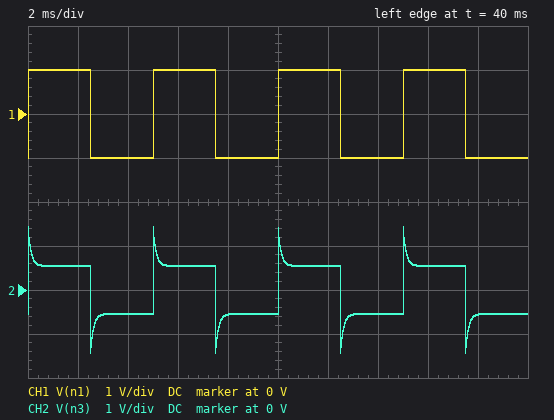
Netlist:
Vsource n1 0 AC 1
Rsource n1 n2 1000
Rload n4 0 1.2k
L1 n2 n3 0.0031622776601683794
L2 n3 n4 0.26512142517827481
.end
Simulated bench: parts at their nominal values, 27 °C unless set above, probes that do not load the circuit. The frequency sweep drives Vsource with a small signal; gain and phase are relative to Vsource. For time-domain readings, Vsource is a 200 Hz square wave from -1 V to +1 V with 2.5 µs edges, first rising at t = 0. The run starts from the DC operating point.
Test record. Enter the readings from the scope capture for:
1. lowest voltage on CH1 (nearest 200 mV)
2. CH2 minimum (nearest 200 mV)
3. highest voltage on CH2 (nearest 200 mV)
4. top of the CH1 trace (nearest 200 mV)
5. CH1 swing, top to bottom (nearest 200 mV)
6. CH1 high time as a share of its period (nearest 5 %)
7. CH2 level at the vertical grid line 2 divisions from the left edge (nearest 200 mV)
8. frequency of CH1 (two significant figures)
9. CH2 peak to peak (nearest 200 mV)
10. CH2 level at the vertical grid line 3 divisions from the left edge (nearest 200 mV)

-1.0 V
-1.4 V
1.4 V
1.0 V
2.0 V
50 %
-600 mV
200 Hz
2.8 V
600 mV
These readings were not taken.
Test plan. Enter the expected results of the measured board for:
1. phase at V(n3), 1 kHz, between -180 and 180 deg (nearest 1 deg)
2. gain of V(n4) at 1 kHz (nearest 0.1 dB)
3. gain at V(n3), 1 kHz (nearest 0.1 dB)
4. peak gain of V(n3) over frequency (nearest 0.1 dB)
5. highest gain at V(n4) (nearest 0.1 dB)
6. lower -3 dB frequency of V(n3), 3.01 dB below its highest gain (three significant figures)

17 deg
-7.3 dB
-2.6 dB
-0.1 dB
-5.3 dB
816 Hz
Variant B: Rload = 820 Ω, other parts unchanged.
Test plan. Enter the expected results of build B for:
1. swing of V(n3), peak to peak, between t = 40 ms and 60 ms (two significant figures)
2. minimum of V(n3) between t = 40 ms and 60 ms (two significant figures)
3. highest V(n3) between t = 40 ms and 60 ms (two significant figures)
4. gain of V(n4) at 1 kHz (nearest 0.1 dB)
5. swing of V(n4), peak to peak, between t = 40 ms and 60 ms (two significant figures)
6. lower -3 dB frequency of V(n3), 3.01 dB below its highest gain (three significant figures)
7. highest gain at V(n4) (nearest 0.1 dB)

3.0 V
-1.5 V
1.5 V
-9.6 dB
900 mV
825 Hz
-6.9 dB
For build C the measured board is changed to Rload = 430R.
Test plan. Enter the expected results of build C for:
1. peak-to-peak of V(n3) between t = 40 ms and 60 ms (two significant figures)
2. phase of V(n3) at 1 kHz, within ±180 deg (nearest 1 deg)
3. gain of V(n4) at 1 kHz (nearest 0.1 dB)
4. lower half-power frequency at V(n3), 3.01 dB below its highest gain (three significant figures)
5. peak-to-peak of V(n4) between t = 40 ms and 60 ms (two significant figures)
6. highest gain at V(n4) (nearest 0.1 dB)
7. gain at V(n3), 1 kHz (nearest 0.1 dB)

3.3 V
26 deg
-14.2 dB
766 Hz
600 mV
-10.4 dB
-2.2 dB
